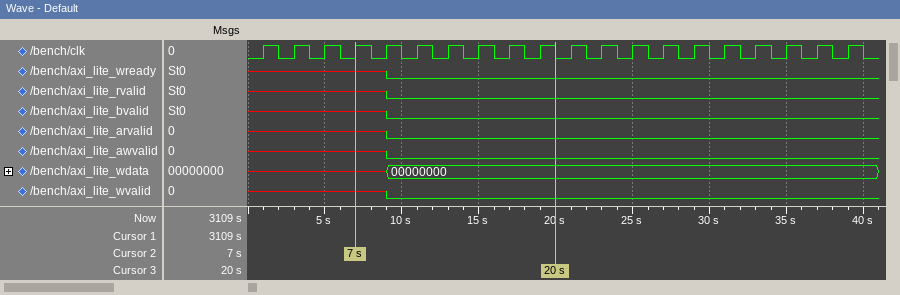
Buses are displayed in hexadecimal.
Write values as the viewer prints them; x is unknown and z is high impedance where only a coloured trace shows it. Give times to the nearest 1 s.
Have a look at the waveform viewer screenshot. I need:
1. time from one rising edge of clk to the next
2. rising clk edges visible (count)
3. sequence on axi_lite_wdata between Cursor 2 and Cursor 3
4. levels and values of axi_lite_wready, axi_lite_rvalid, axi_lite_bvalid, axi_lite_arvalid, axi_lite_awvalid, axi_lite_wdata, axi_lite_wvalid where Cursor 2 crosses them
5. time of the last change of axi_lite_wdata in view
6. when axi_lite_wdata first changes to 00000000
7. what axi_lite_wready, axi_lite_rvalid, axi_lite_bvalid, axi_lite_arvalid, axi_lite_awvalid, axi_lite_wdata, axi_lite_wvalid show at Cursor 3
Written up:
2 s
20
x, 00000000
axi_lite_wready=x, axi_lite_rvalid=x, axi_lite_bvalid=x, axi_lite_arvalid=x, axi_lite_awvalid=x, axi_lite_wdata=x, axi_lite_wvalid=x
9 s
9 s
axi_lite_wready=0, axi_lite_rvalid=0, axi_lite_bvalid=0, axi_lite_arvalid=0, axi_lite_awvalid=0, axi_lite_wdata=00000000, axi_lite_wvalid=0
